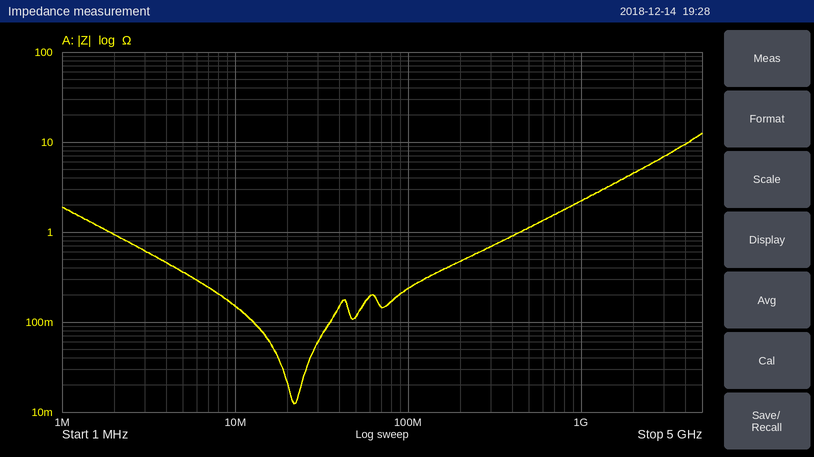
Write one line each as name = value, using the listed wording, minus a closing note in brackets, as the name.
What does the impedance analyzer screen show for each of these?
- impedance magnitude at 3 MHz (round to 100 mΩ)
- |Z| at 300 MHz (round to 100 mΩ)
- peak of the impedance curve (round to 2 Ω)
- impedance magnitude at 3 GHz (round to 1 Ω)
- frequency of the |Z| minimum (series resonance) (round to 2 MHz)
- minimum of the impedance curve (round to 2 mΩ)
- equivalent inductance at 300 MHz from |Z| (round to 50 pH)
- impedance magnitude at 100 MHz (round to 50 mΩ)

impedance magnitude at 3 MHz = 600 mΩ
|Z| at 300 MHz = 700 mΩ
peak of the impedance curve = 12 Ω
impedance magnitude at 3 GHz = 7 Ω
frequency of the |Z| minimum (series resonance) = 22 MHz
minimum of the impedance curve = 12 mΩ
equivalent inductance at 300 MHz from |Z| = 350 pH
impedance magnitude at 100 MHz = 250 mΩ
